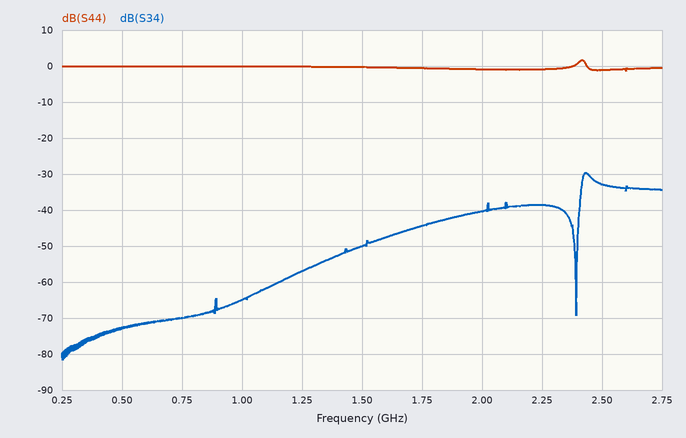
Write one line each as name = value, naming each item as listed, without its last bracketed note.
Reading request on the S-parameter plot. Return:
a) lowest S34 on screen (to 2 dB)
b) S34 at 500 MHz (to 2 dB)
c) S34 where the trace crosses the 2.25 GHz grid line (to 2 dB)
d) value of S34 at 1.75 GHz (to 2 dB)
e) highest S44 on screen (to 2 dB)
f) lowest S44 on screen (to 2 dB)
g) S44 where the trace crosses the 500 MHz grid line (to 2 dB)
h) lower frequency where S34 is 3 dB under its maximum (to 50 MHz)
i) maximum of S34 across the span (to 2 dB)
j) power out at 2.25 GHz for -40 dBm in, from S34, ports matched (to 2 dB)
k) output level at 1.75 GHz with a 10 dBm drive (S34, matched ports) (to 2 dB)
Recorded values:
lowest S34 on screen = -82 dB
S34 at 500 MHz = -72 dB
S34 where the trace crosses the 2.25 GHz grid line = -38 dB
value of S34 at 1.75 GHz = -44 dB
highest S44 on screen = 2 dB
lowest S44 on screen = -2 dB
S44 where the trace crosses the 500 MHz grid line = 0 dB
lower frequency where S34 is 3 dB under its maximum = 2.40 GHz
maximum of S34 across the span = -30 dB
power out at 2.25 GHz for -40 dBm in, from S34, ports matched = -78 dBm
output level at 1.75 GHz with a 10 dBm drive (S34, matched ports) = -34 dBm
